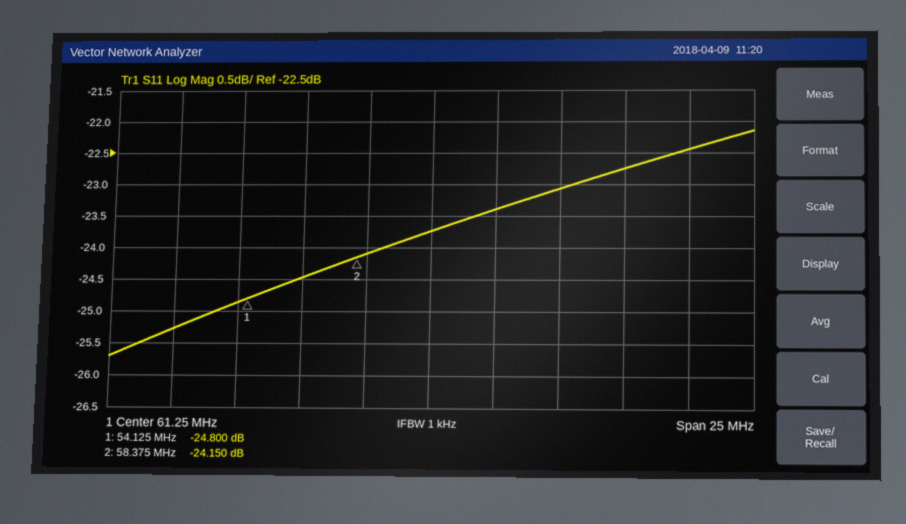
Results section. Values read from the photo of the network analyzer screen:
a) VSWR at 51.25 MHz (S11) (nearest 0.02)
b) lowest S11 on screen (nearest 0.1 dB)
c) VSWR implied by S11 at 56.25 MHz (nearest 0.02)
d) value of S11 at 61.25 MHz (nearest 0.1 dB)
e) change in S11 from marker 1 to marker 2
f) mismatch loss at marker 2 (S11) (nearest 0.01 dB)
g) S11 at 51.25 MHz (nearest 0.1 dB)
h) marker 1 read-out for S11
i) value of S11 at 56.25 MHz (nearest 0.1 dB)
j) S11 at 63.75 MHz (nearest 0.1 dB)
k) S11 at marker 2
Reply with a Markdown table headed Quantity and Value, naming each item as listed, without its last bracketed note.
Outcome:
| Quantity | Value |
|---|---|
| VSWR at 51.25 MHz (S11) | 1.12 |
| lowest S11 on screen | -25.7 dB |
| VSWR implied by S11 at 56.25 MHz | 1.12 |
| value of S11 at 61.25 MHz | -23.7 dB |
| change in S11 from marker 1 to marker 2 | 0.650 dB |
| mismatch loss at marker 2 (S11) | 0.02 dB |
| S11 at 51.25 MHz | -25.3 dB |
| marker 1 read-out for S11 | -24.800 dB |
| value of S11 at 56.25 MHz | -24.5 dB |
| S11 at 63.75 MHz | -23.4 dB |
| S11 at marker 2 | -24.150 dB |
